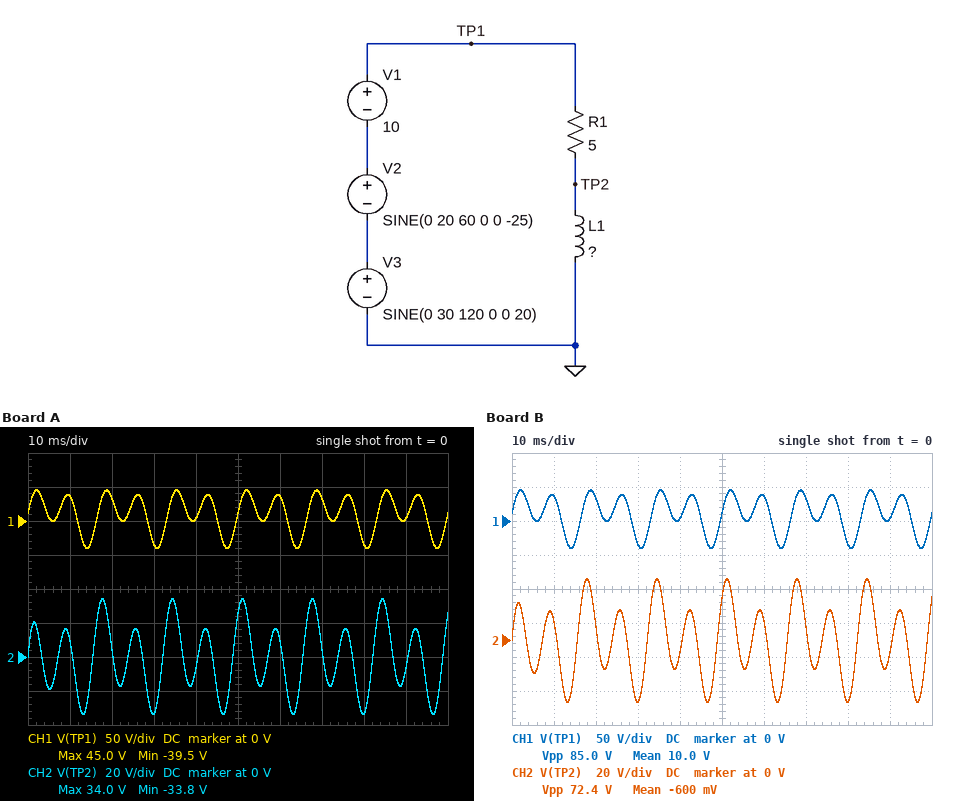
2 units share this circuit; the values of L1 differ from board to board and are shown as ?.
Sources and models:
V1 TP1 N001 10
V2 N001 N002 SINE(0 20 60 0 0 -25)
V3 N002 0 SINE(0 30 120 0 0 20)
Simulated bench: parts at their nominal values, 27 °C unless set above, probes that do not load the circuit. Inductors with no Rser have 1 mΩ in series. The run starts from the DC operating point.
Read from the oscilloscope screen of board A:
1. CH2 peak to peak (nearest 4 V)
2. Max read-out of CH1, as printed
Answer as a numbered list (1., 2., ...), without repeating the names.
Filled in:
1. 68 V
2. 45.0 V
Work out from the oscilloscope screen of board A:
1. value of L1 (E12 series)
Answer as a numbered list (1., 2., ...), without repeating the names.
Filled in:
1. 10 mH
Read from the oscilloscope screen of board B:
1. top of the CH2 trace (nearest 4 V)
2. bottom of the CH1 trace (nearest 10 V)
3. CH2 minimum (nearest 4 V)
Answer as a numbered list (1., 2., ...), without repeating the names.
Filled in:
1. 36 V
2. -40 V
3. -36 V
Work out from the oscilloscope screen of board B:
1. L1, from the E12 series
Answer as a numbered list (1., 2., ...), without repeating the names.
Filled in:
1. 12 mH
